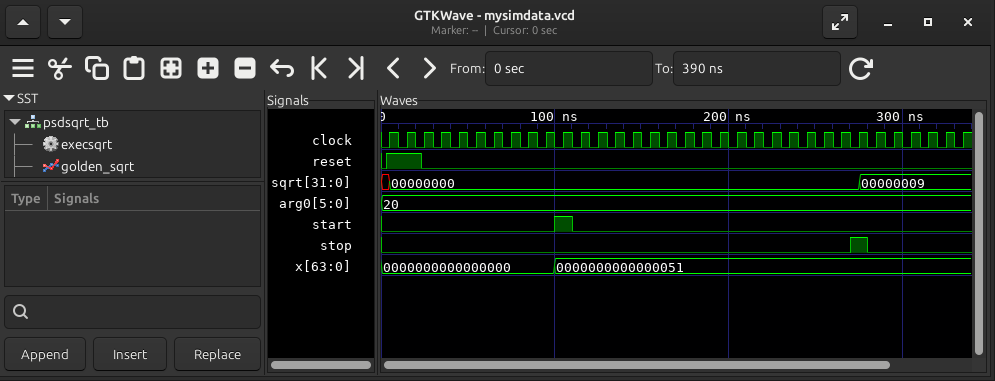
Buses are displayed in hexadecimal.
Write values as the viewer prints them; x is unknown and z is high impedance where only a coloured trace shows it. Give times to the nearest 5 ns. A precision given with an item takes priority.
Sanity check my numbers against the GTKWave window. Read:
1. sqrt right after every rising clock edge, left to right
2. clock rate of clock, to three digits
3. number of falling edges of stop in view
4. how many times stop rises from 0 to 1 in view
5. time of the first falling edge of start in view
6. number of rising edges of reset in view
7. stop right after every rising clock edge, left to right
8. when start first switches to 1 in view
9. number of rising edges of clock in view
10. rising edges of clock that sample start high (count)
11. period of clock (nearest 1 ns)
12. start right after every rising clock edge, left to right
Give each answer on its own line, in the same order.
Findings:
00000000, 00000000, 00000000, 00000000, 00000000, 00000000, 00000000, 00000000, 00000000, 00000000, 00000000, 00000000, 00000000, 00000000, 00000000, 00000000, 00000000, 00000000, 00000000, 00000000, 00000000, 00000000, 00000000, 00000000, 00000000, 00000000, 00000000, 00000009, 00000009, 00000009, 00000009, 00000009, 00000009, 00000009
100 MHz
1
1
110 ns
1
0 0 0 0 0 0 0 0 0 0 0 0 0 0 0 0 0 0 0 0 0 0 0 0 0 0 0 1 0 0 0 0 0 0
100 ns
34
1
10 ns
0 0 0 0 0 0 0 0 0 0 1 0 0 0 0 0 0 0 0 0 0 0 0 0 0 0 0 0 0 0 0 0 0 0
